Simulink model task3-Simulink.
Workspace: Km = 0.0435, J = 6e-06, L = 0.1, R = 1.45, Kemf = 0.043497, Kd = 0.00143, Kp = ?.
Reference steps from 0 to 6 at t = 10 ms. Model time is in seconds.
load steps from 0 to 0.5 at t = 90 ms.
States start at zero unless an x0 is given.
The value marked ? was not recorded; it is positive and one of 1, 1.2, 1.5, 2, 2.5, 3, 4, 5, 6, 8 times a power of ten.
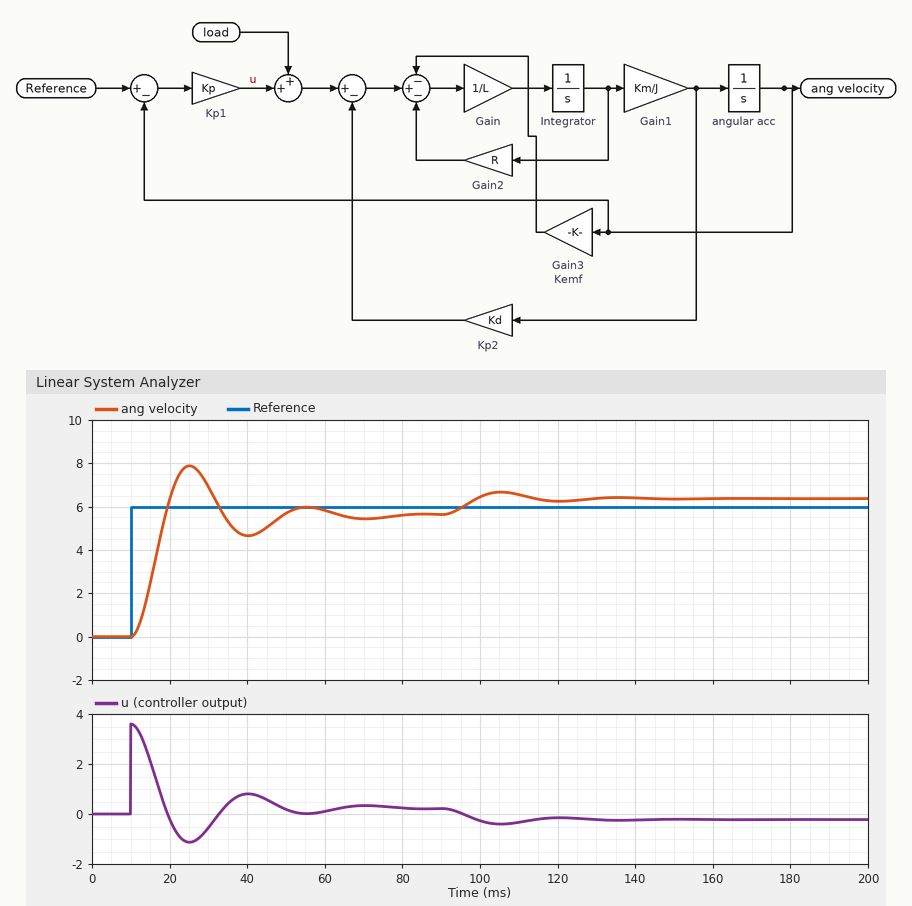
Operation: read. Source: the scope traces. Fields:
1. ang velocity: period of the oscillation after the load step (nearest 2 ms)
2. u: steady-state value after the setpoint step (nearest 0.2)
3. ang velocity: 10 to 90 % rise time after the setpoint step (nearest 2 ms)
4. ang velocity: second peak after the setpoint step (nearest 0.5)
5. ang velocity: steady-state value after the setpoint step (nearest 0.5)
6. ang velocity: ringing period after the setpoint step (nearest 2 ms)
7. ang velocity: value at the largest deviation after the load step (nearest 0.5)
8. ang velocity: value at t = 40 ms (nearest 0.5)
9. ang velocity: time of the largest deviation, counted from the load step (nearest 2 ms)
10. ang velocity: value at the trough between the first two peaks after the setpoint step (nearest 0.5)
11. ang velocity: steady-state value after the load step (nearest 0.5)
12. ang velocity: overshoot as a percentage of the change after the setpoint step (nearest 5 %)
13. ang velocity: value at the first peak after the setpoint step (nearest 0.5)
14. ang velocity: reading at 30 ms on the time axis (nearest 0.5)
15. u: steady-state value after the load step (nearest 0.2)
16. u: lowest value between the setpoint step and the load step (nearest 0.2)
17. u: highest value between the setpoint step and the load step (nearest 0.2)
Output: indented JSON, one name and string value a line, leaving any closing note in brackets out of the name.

{
  "ang velocity: period of the oscillation after the load step": "30 ms",
  "u: steady-state value after the setpoint step": "0.2",
  "ang velocity: 10 to 90 % rise time after the setpoint step": "6 ms",
  "ang velocity: second peak after the setpoint step": "6.0",
  "ang velocity: steady-state value after the setpoint step": "5.5",
  "ang velocity: ringing period after the setpoint step": "30 ms",
  "ang velocity: value at the largest deviation after the load step": "6.5",
  "ang velocity: value at t = 40 ms": "4.5",
  "ang velocity: time of the largest deviation, counted from the load step": "16 ms",
  "ang velocity: value at the trough between the first two peaks after the setpoint step": "4.5",
  "ang velocity: steady-state value after the load step": "6.5",
  "ang velocity: overshoot as a percentage of the change after the setpoint step": "40 %",
  "ang velocity: value at the first peak after the setpoint step": "8.0",
  "ang velocity: reading at 30 ms on the time axis": "7.0",
  "u: steady-state value after the load step": "-0.2",
  "u: lowest value between the setpoint step and the load step": "-1.2",
  "u: highest value between the setpoint step and the load step": "3.6"
}
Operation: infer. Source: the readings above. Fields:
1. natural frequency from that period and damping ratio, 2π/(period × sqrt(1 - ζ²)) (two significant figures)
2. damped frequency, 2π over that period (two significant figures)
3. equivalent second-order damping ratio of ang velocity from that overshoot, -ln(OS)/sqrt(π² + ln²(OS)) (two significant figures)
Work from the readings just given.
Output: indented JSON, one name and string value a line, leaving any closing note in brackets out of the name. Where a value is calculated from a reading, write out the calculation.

{
  "natural frequency from that period and damping ratio, 2π/(period × sqrt(1 - ζ²))": "2π / (30 × sqrt(1 - 0.28²)) = 0.22 rad/ms",
  "damped frequency, 2π over that period": "2π / 30 = 0.21 rad/ms",
  "equivalent second-order damping ratio of ang velocity from that overshoot, -ln(OS)/sqrt(π² + ln²(OS))": "ln(0.4) = -0.916; 0.916 / sqrt(9.870 + 0.840) = 0.28"
}
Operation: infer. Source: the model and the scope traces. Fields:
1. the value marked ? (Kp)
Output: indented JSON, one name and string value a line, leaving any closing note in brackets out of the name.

{
  "the value marked ?": "0.6"
}
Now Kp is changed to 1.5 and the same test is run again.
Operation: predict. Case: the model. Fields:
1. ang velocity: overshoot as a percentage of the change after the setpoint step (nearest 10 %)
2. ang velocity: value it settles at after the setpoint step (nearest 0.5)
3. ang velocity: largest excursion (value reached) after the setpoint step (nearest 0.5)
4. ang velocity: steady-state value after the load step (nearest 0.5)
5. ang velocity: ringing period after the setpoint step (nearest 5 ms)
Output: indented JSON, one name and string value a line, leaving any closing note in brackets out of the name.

{
  "ang velocity: overshoot as a percentage of the change after the setpoint step": "60 %",
  "ang velocity: value it settles at after the setpoint step": "6.0",
  "ang velocity: largest excursion (value reached) after the setpoint step": "9.0",
  "ang velocity: steady-state value after the load step": "6.0",
  "ang velocity: ringing period after the setpoint step": "20 ms"
}
